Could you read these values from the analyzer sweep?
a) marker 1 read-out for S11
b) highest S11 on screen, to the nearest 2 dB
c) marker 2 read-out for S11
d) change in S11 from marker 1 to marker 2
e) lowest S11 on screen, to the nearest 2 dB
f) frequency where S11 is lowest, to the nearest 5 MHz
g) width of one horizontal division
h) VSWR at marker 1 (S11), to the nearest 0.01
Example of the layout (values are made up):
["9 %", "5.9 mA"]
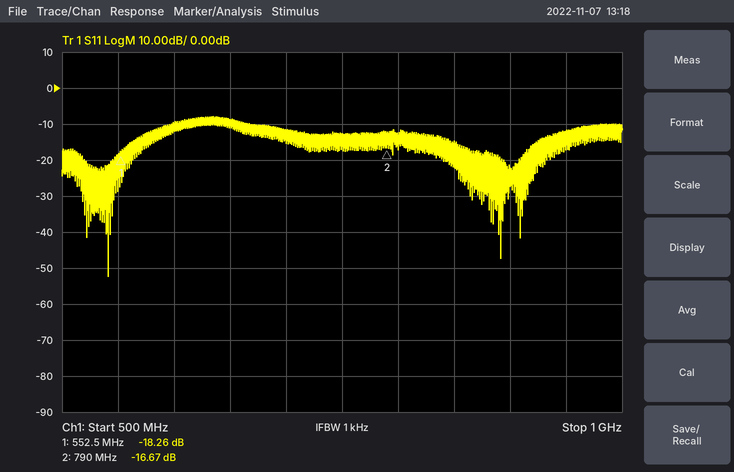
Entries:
["-18.26 dB", "-8 dB", "-16.67 dB", "1.59 dB", "-52 dB", "540 MHz", "50 MHz", "1.28"]
